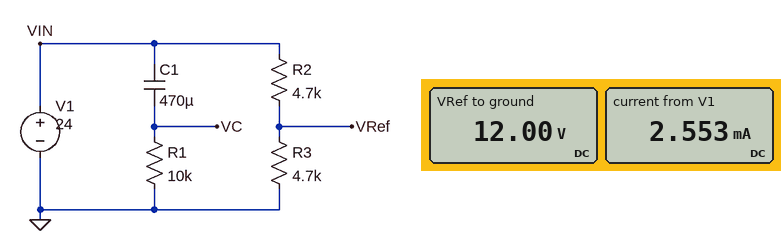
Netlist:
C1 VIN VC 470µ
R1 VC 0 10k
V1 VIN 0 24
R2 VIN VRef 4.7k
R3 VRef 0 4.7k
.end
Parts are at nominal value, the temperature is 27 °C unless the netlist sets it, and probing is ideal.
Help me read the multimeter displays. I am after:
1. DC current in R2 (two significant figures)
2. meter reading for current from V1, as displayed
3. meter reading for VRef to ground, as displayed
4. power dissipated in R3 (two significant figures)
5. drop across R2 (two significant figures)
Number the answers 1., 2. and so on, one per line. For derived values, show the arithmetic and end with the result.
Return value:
1. (24 V - 12 V) / 4.7 kΩ = 2.6 mA
2. 2.553 mA
3. 12.00 V
4. (12 V)^2 / 4.7 kΩ = 31 mW
5. 24 V - 12 V = 12 V
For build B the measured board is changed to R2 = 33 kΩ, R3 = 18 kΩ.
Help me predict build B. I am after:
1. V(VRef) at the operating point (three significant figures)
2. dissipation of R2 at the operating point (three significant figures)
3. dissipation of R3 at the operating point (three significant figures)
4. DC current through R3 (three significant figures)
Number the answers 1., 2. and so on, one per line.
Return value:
1. 8.47 V
2. 7.31 mW
3. 3.99 mW
4. 471 µA
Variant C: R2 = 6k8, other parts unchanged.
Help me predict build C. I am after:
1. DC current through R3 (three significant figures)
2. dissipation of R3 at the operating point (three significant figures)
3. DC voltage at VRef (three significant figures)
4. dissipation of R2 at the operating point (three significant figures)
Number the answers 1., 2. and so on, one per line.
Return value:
1. 2.09 mA
2. 20.5 mW
3. 9.81 V
4. 29.6 mW
